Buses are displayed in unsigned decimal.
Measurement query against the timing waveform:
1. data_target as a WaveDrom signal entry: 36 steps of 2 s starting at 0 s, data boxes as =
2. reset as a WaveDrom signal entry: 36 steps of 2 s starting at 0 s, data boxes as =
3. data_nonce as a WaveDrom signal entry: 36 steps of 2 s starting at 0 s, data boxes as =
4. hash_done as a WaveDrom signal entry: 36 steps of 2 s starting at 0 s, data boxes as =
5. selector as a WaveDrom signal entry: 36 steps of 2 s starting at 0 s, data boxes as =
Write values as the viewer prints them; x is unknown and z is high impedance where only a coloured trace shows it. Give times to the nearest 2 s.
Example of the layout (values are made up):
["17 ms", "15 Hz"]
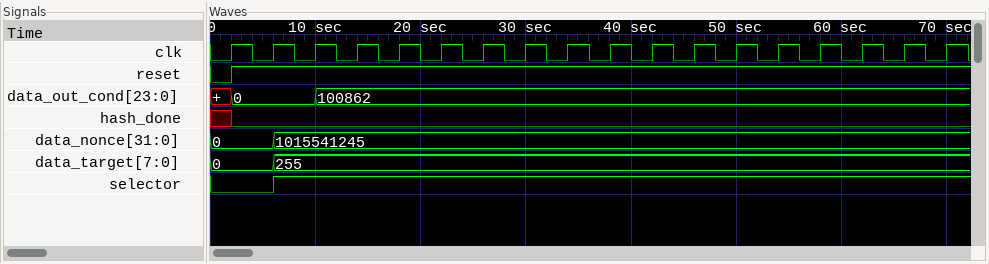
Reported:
["{name: 'data_target', wave: '=..=................................', data: '0 255'}", "{name: 'reset', wave: '01..................................'}", "{name: 'data_nonce', wave: '=..=................................', data: '0 1015541245'}", "{name: 'hash_done', wave: 'x0..................................'}", "{name: 'selector', wave: '0..1................................'}"]
